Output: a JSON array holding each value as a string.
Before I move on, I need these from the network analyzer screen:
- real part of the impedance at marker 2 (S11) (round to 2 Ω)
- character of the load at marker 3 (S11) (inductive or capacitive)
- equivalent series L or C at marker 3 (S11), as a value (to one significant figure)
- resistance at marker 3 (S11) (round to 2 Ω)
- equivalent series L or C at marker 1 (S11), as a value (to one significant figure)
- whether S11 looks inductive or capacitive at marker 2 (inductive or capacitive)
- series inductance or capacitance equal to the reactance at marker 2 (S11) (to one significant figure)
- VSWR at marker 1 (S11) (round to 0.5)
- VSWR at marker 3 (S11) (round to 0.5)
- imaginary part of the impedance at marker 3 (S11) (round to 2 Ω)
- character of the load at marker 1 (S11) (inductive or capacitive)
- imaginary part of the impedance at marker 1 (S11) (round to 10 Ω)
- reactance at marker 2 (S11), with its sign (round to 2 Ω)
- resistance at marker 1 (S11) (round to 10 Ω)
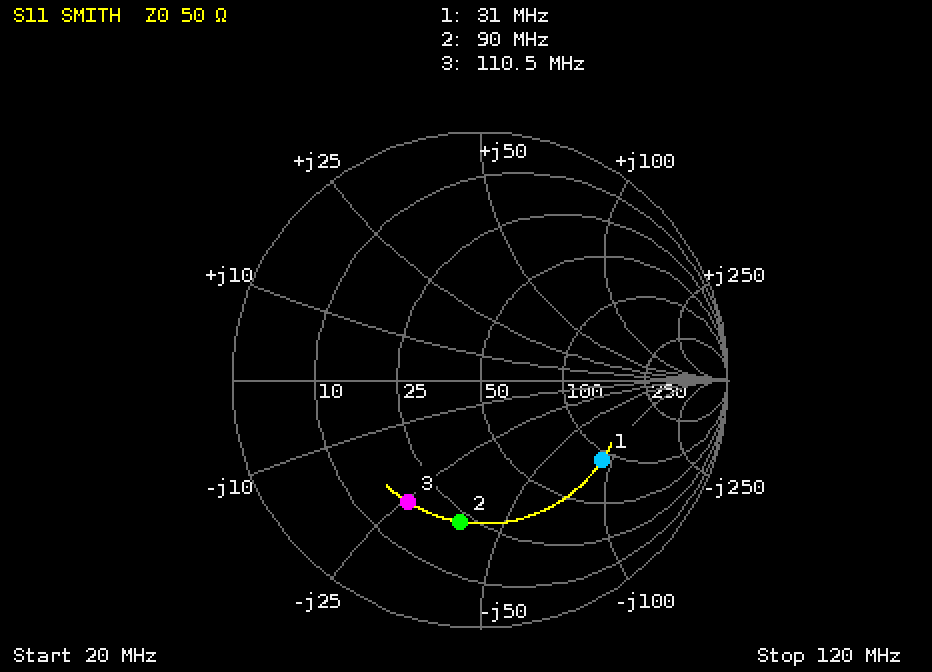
["22 Ω", "capacitive", "60 pF", "18 Ω", "60 pF", "capacitive", "50 pF", "4.0", "3.5", "-26 Ω", "capacitive", "-90 Ω", "-38 Ω", "90 Ω"]
